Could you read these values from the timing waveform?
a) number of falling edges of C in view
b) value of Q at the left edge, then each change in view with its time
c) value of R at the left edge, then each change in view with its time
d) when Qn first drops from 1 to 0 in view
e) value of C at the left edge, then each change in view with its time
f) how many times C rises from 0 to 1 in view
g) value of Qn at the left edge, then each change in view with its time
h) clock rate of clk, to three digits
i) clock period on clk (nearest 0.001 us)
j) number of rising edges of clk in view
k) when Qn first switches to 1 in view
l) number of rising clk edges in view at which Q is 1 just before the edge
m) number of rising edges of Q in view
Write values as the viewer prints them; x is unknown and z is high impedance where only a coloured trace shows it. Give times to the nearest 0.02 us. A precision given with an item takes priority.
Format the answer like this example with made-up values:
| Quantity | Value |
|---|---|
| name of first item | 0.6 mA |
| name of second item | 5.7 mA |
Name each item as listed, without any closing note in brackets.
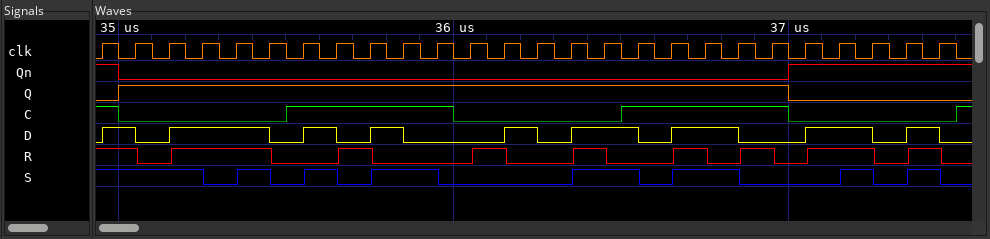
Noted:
| Quantity | Value |
|---|---|
| number of falling edges of C in view | 3 |
| value of Q at the left edge, then each change in view with its time | 0, 1 at 35 us, 0 at 37 us |
| value of R at the left edge, then each change in view with its time | 1, 0 at 35.06 us, 1 at 35.16 us, 0 at 35.46 us, 1 at 35.66 us, 0 at 35.76 us, 1 at 36.06 us, 0 at 36.16 us, 1 at 36.36 us, 0 at 36.46 us, 1 at 36.66 us, 0 at 36.76 us, 1 at 36.86 us, 0 at 36.96 us, 1 at 37.06 us, 0 at 37.26 us, 1 at 37.36 us, 0 at 37.46 us |
| when Qn first drops from 1 to 0 in view | 35 us |
| value of C at the left edge, then each change in view with its time | 1, 0 at 35 us, 1 at 35.5 us, 0 at 36 us, 1 at 36.5 us, 0 at 37 us, 1 at 37.5 us |
| how many times C rises from 0 to 1 in view | 3 |
| value of Qn at the left edge, then each change in view with its time | 1, 0 at 35 us, 1 at 37 us |
| clock rate of clk, to three digits | 10.0 MHz |
| clock period on clk | 0.1 us |
| number of rising edges of clk in view | 26 |
| when Qn first switches to 1 in view | 37 us |
| number of rising clk edges in view at which Q is 1 just before the edge | 20 |
| number of rising edges of Q in view | 1 |
